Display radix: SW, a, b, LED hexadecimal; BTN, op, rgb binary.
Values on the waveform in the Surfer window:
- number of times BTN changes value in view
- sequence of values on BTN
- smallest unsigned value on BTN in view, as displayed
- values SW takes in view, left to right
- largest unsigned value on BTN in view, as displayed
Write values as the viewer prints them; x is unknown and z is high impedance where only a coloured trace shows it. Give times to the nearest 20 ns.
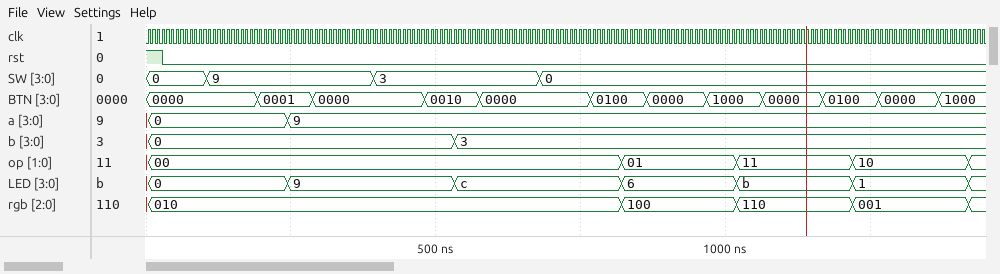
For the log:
11
0000, 0001, 0000, 0010, 0000, 0100, 0000, 1000, 0000, 0100, 0000, 1000
0000
0, 9, 3, 0
1000
